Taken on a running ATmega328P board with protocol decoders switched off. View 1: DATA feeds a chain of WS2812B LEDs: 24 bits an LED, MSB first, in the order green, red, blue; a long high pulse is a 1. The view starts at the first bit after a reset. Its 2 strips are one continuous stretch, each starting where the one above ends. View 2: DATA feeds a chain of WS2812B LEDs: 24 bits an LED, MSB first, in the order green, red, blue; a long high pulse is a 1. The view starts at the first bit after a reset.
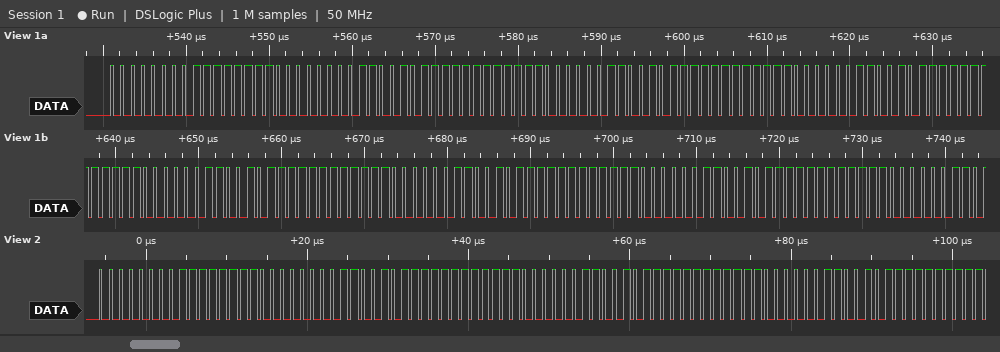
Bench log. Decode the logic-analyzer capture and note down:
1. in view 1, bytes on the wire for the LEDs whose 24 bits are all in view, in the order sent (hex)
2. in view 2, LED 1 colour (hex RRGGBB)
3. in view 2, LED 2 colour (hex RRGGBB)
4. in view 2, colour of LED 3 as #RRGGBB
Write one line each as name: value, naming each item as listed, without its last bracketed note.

in view 1, bytes on the wire for the LEDs whose 24 bits are all in view, in the order sent: 00 FF 00 CB FF C0 CB FF C0 CB FF C0 CB FF C0 CB FF C0 CB FF C0
in view 2, LED 1 colour: #FF0000
in view 2, LED 2 colour: #FFCBC0
in view 2, colour of LED 3 as #RRGGBB: #FFCBC0
